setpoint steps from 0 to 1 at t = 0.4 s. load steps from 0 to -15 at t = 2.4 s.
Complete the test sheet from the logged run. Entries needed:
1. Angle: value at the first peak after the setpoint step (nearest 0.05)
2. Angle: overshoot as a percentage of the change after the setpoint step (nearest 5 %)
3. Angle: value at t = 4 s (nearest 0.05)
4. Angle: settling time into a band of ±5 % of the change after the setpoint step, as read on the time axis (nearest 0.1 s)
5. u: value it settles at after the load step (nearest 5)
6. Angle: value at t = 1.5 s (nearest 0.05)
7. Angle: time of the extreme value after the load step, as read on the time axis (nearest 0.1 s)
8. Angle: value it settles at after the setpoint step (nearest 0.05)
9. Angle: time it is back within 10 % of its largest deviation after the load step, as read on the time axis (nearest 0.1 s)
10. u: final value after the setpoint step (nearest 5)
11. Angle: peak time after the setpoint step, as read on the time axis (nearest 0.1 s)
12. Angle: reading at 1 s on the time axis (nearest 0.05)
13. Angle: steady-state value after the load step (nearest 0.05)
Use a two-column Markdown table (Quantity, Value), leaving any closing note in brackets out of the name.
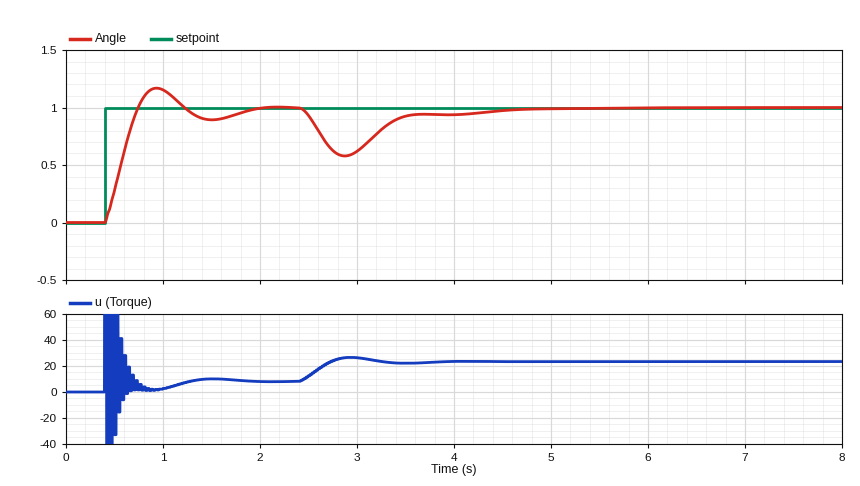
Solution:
| Quantity | Value |
|---|---|
| Angle: value at the first peak after the setpoint step | 1.15 |
| Angle: overshoot as a percentage of the change after the setpoint step | 15 % |
| Angle: value at t = 4 s | 0.95 |
| Angle: settling time into a band of ±5 % of the change after the setpoint step, as read on the time axis | 1.8 s |
| u: value it settles at after the load step | 25 |
| Angle: value at t = 1.5 s | 0.90 |
| Angle: time of the extreme value after the load step, as read on the time axis | 2.9 s |
| Angle: value it settles at after the setpoint step | 1.00 |
| Angle: time it is back within 10 % of its largest deviation after the load step, as read on the time axis | 4.3 s |
| u: final value after the setpoint step | 10 |
| Angle: peak time after the setpoint step, as read on the time axis | 0.9 s |
| Angle: reading at 1 s on the time axis | 1.15 |
| Angle: steady-state value after the load step | 1.00 |
